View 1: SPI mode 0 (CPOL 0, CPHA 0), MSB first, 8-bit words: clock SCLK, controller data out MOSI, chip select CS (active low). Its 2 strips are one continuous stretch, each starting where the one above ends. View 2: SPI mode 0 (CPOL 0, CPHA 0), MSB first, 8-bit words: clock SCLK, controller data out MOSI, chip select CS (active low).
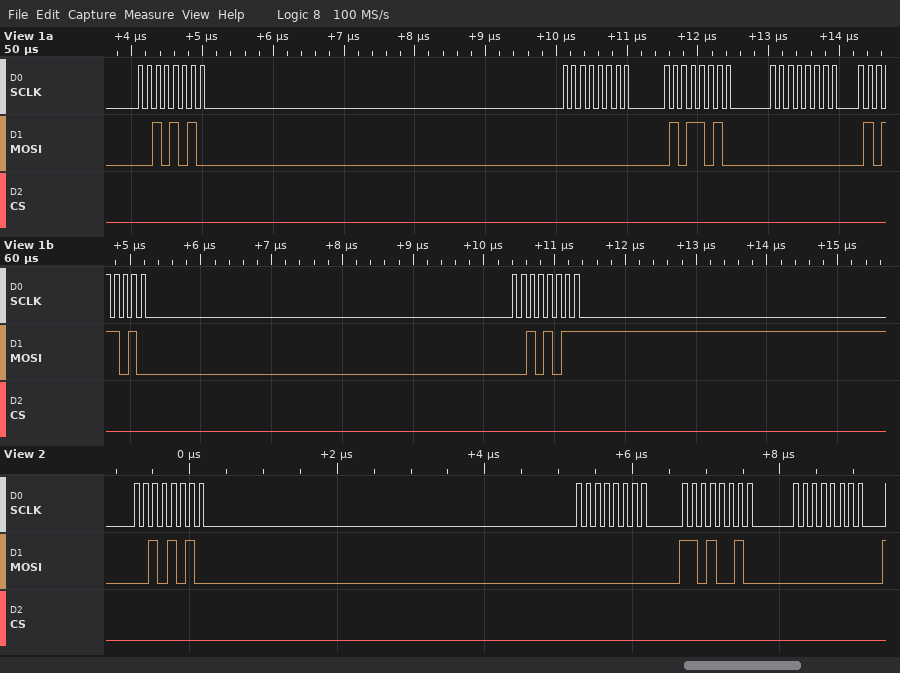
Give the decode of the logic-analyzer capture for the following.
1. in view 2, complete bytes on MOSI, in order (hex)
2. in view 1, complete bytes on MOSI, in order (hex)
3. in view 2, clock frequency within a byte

2A 00 D2 00
2A 00 5A 00 5A 2B
8 MHz
